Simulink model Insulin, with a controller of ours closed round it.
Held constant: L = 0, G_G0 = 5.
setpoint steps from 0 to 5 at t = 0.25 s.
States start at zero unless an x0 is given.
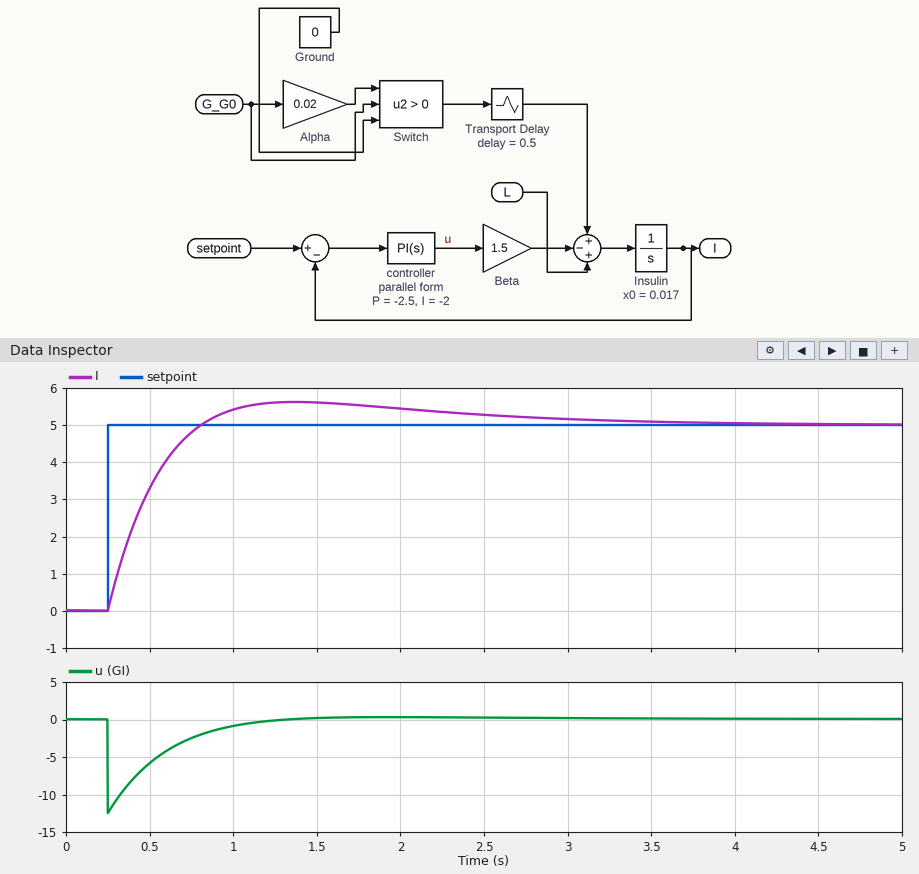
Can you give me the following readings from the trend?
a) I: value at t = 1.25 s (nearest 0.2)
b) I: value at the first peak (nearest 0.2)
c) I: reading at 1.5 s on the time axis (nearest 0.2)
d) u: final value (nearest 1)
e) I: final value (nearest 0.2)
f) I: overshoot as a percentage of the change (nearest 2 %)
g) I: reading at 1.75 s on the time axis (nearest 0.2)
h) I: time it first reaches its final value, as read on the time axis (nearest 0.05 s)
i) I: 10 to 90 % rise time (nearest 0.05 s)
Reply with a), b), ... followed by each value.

a) 5.6
b) 5.6
c) 5.6
d) 0
e) 5.0
f) 12 %
g) 5.6
h) 0.80 s
i) 0.40 s
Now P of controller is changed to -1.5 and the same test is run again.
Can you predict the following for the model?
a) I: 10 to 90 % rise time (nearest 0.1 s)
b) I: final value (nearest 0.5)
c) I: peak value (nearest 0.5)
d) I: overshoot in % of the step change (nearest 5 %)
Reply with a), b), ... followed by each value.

a) 0.5 s
b) 5.0
c) 6.0
d) 25 %
